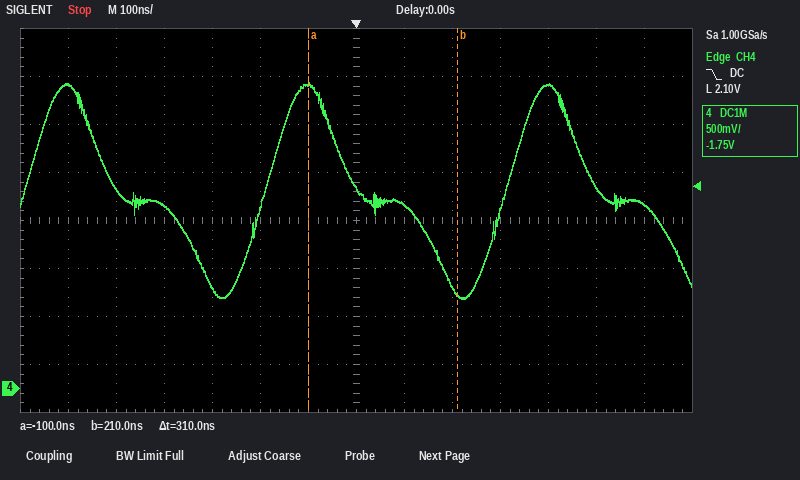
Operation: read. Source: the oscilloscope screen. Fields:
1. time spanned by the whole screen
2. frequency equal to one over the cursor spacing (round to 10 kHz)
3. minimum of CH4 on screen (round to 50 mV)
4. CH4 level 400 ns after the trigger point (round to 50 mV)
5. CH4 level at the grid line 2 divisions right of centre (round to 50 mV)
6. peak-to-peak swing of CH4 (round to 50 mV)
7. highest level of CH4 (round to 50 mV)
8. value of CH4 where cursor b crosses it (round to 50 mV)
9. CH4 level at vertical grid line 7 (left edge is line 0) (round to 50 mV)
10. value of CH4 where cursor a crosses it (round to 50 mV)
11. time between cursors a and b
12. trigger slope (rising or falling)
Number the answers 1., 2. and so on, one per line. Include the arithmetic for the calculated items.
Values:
1. 1.4 µs
2. 1 / 310 ns ≈ 3.23 MHz
3. 950 mV
4. 3.15 V
5. 1.05 V
6. 3.20 V − (950 mV) = 2.25 V
7. 3.20 V
8. 1.00 V
9. 2.10 V
10. 3.15 V
11. 310 ns
12. falling
